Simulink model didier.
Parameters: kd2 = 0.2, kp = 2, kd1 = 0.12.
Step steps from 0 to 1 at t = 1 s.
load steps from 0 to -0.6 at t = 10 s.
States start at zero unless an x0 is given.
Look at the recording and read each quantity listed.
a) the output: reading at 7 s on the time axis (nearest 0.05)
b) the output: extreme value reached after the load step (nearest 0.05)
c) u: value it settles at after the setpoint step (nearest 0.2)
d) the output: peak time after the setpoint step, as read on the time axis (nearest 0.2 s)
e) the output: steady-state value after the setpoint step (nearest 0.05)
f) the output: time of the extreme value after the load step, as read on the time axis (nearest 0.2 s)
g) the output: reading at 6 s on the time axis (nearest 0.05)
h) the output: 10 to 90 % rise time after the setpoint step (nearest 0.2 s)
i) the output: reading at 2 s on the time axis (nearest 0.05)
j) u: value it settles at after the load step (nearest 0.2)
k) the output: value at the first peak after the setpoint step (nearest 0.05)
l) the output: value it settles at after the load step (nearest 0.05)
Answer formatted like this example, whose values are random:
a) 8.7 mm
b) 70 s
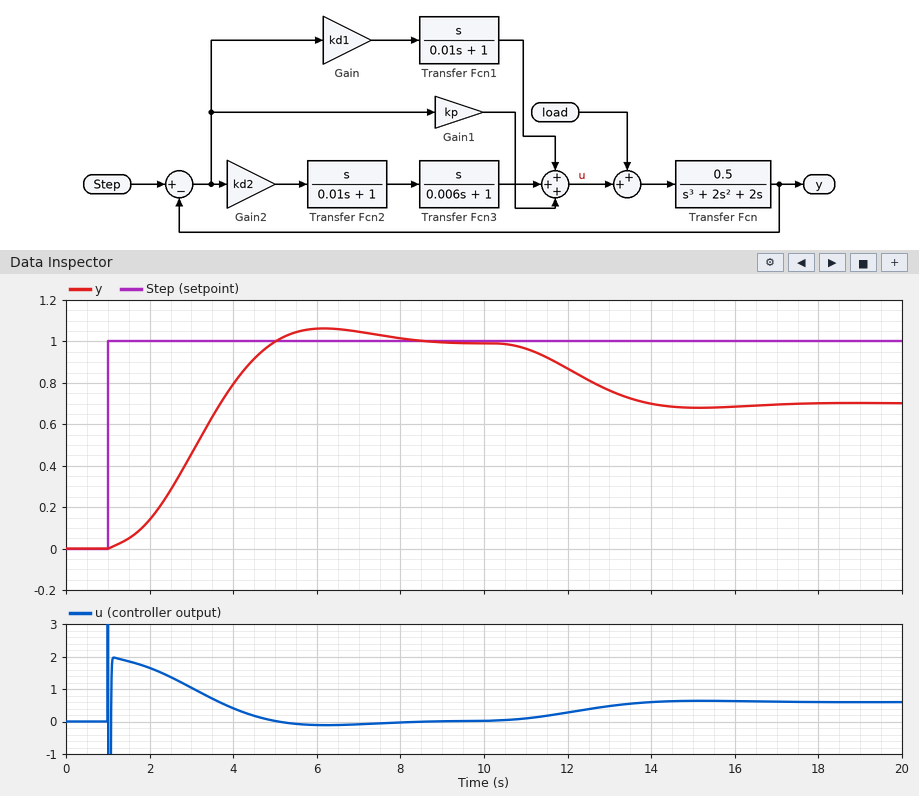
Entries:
a) 1.05
b) 0.70
c) 0.0
d) 6.2 s
e) 1.00
f) 15.2 s
g) 1.05
h) 2.6 s
i) 0.15
j) 0.6
k) 1.05
l) 0.70
